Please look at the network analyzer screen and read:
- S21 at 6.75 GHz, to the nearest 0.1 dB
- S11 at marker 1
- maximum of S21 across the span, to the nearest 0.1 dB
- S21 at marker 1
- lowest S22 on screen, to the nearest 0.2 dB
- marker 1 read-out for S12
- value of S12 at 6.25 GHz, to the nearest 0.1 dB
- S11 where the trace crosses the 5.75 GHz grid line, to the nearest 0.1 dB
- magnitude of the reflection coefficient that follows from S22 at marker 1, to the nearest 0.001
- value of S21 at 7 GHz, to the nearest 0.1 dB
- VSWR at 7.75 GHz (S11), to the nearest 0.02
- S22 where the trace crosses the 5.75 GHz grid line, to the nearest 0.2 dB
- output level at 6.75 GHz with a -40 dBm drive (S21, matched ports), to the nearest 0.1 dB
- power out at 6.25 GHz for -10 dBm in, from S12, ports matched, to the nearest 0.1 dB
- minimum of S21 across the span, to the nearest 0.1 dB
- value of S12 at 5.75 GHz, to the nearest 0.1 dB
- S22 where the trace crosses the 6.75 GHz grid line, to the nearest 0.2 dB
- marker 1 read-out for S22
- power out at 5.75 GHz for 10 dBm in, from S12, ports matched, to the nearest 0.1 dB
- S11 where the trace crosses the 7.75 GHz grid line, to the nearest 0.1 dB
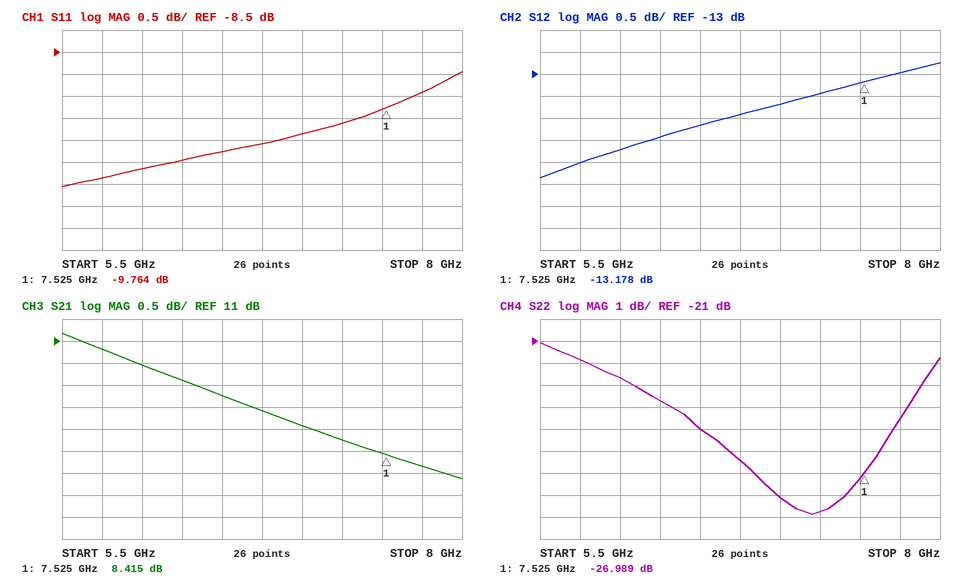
9.4 dB
-9.764 dB
11.2 dB
8.415 dB
-28.8 dB
-13.178 dB
-14.4 dB
-11.4 dB
0.045
9.1 dB
2.02
-21.8 dB
-30.6 dBm
-24.4 dBm
7.9 dB
-15.0 dB
-26.4 dB
-26.989 dB
-5.0 dBm
-9.4 dB
